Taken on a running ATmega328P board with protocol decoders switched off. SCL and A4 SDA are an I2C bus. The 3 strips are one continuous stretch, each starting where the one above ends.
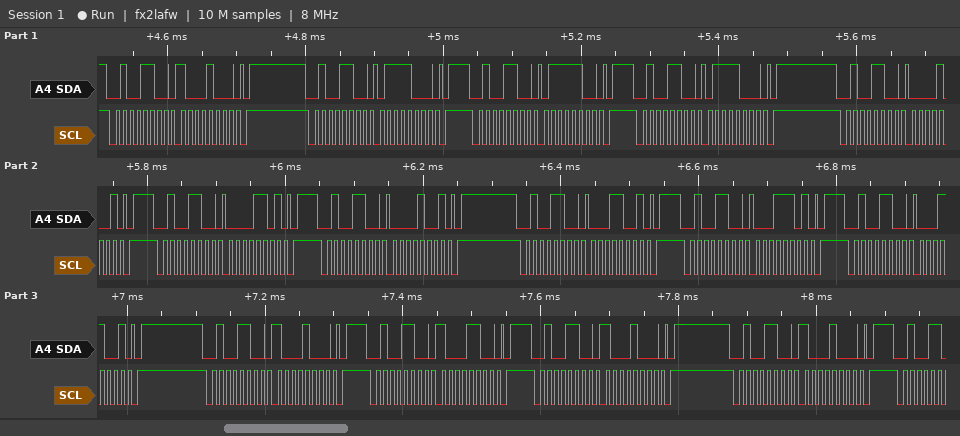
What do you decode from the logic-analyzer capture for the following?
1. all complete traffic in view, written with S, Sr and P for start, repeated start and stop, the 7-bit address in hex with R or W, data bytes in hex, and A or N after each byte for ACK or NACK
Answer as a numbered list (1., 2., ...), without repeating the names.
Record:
1. S 26W A 88 A P S 26W A 78 A P S 26W A 7C A P S 26W A 78 A P S 26W A 09 A P S 26W A 0D A P S 26W A 09 A P S 26W A 19 A P S 26W A 1D A P S 26W A 19 A P S 26W A 88 A P S 26W A 8C A P S 26W A 88 A P S 26W A 88 A P
